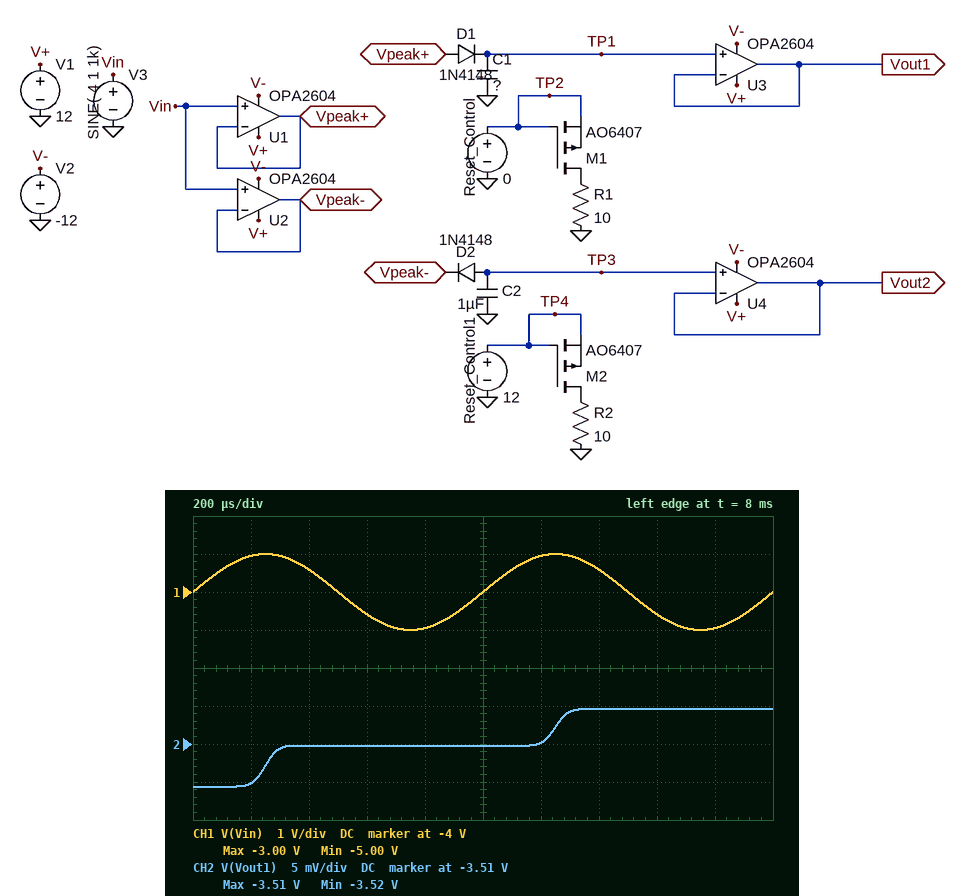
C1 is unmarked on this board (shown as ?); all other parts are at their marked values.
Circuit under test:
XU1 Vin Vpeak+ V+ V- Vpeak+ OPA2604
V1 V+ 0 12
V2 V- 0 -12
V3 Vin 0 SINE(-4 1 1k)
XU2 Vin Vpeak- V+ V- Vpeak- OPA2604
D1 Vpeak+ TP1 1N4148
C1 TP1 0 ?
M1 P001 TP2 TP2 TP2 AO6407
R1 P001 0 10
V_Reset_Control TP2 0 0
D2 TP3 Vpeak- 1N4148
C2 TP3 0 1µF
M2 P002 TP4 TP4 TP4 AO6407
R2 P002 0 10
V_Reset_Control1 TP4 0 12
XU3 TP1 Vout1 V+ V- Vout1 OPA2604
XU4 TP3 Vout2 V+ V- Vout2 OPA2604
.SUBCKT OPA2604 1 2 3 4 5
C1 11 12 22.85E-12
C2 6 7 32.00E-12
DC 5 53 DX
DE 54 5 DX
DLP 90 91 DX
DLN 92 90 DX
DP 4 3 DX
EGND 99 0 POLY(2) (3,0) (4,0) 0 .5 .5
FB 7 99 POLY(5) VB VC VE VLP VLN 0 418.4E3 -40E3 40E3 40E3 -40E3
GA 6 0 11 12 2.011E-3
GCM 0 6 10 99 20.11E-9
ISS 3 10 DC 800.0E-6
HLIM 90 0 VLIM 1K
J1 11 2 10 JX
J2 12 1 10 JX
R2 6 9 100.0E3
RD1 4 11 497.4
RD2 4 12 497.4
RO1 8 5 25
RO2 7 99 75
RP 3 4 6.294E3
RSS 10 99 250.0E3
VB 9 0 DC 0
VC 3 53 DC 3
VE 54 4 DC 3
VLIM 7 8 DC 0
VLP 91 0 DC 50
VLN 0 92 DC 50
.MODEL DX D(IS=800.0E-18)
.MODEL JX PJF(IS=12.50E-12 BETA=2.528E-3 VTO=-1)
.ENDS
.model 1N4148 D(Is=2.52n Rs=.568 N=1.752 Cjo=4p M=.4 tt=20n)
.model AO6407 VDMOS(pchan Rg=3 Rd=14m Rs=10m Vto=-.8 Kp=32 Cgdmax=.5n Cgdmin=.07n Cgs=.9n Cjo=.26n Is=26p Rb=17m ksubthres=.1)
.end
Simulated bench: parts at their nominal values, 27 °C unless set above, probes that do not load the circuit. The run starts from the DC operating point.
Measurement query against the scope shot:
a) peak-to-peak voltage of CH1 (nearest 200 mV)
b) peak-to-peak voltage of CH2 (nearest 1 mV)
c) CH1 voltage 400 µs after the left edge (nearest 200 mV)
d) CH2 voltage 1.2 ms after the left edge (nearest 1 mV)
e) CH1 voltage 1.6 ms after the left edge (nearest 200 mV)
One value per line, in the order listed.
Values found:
2.0 V
10 mV
-3.4 V
-3.510 V
-4.6 V
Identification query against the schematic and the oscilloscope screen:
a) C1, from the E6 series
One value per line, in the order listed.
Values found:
3.3 µF
